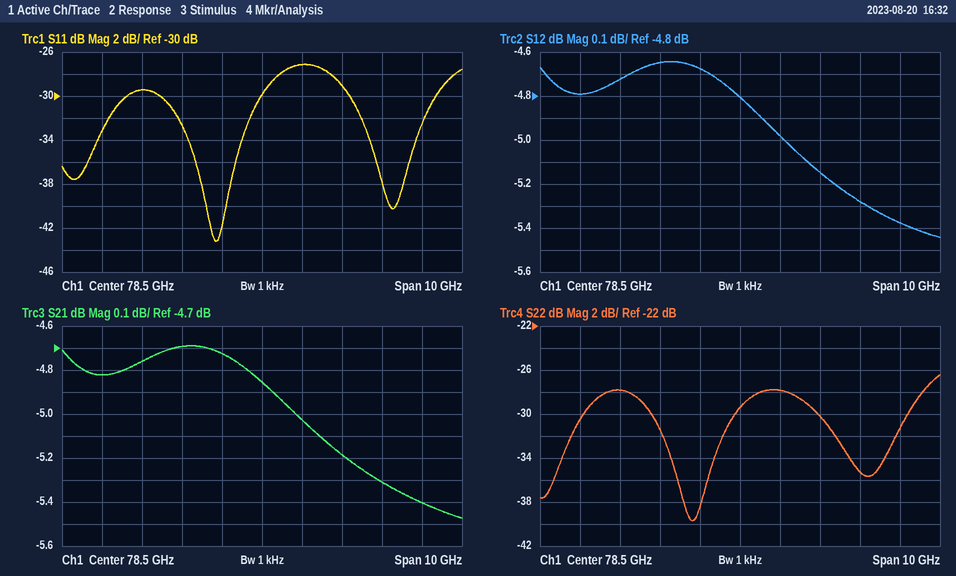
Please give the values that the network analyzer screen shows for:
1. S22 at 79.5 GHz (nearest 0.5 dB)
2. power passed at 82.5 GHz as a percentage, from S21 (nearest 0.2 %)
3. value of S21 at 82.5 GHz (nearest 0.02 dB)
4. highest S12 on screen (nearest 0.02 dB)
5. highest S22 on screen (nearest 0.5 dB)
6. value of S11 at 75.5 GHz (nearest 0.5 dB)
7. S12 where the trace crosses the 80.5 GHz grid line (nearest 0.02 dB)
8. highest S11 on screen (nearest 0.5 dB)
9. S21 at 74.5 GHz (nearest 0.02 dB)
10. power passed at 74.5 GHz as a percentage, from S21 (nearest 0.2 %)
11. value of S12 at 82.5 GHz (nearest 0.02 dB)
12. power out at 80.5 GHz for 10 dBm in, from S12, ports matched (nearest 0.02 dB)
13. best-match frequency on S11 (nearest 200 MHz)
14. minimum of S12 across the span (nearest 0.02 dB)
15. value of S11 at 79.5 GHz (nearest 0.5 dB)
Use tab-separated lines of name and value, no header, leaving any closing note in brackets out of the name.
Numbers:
S22 at 79.5 GHz	-28.0 dB
power passed at 82.5 GHz as a percentage, from S21	28.8 %
value of S21 at 82.5 GHz	-5.40 dB
highest S12 on screen	-4.64 dB
highest S22 on screen	-26.5 dB
value of S11 at 75.5 GHz	-29.5 dB
S12 where the trace crosses the 80.5 GHz grid line	-5.14 dB
highest S11 on screen	-27.0 dB
S21 at 74.5 GHz	-4.82 dB
power passed at 74.5 GHz as a percentage, from S21	33.0 %
value of S12 at 82.5 GHz	-5.38 dB
power out at 80.5 GHz for 10 dBm in, from S12, ports matched	4.86 dBm
best-match frequency on S11	77.4 GHz
minimum of S12 across the span	-5.44 dB
value of S11 at 79.5 GHz	-27.0 dB
